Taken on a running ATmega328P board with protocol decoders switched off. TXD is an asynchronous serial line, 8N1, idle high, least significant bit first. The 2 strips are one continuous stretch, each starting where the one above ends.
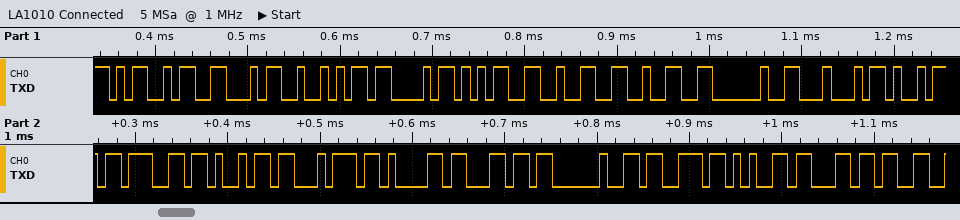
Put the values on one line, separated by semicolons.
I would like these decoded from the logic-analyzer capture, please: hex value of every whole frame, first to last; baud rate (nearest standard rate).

4D 46 52 43 35 32 32 20 44 69 67 69 74 61 6C 20 73 65 6C; 115200 baud
